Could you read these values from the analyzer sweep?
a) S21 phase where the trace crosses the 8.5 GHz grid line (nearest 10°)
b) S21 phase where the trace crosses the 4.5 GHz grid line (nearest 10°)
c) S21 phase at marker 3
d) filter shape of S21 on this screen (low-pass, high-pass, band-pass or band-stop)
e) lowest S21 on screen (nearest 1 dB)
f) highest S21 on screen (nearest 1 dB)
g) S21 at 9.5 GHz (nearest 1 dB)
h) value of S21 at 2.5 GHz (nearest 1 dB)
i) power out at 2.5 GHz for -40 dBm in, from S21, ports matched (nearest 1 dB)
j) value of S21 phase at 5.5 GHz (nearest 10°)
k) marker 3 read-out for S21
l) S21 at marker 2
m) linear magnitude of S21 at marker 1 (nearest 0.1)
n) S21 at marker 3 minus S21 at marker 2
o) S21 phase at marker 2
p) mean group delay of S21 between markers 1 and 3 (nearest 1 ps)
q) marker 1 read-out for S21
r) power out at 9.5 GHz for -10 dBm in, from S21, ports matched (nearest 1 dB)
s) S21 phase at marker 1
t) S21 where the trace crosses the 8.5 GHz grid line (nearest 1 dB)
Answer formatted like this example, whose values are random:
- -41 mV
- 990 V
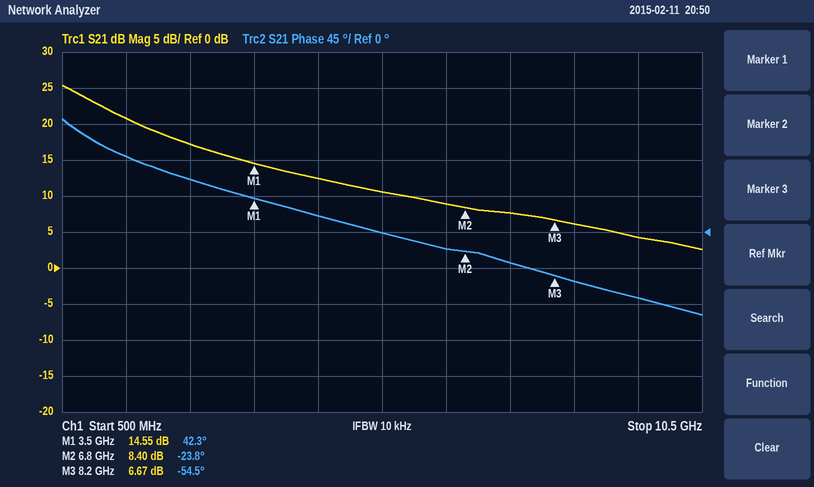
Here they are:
- -60°
- 20°
- -54.5°
- low-pass
- 3 dB
- 25 dB
- 4 dB
- 17 dB
- -23 dBm
- 0°
- 6.67 dB
- 8.40 dB
- 5.3
- -1.73 dB
- -23.8°
- 57 ps
- 14.55 dB
- -6 dBm
- 42.3°
- 6 dB
